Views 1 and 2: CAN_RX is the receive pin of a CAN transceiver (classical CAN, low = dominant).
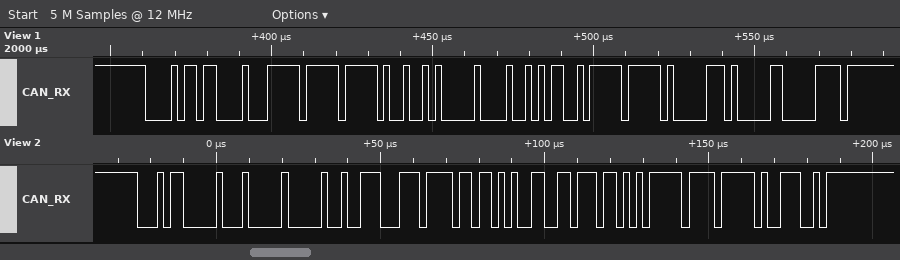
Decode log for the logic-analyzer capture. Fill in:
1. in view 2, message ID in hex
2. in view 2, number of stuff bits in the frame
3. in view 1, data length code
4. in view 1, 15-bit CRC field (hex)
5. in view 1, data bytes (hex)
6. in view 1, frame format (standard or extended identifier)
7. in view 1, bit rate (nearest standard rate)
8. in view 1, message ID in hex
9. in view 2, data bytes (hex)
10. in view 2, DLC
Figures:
0x160
5
8
0x2083
FF FF 25 00 4A CB FF 83
standard
500 kbit/s
0x0B6
00 4E 3B DB 53 37 6A FF
8
